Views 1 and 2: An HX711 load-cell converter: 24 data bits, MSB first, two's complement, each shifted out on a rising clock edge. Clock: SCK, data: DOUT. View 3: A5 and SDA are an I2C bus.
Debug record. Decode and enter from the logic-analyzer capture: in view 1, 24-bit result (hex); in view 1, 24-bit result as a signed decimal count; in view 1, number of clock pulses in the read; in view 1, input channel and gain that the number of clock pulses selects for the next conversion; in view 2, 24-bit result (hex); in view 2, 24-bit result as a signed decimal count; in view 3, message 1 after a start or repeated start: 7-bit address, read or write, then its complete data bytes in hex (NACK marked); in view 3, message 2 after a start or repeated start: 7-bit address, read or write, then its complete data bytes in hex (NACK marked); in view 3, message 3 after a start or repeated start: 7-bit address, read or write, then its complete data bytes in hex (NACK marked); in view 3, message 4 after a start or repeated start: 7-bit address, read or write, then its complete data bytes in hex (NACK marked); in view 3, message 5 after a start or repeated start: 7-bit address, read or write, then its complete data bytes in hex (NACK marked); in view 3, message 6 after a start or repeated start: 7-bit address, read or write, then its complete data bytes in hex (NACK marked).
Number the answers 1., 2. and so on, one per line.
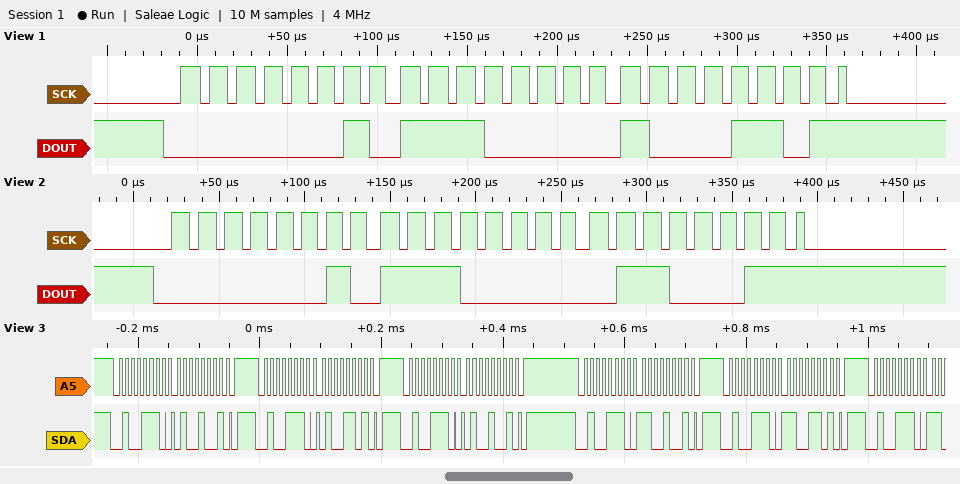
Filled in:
1. 0x02E08D
2. 188557
3. 25
4. channel A, gain 128
5. 0x02E063
6. 188515
7. 0x27 write: 49
8. 0x27 write: 4D
9. 0x27 write: 49
10. 0x27 write: C9
11. 0x27 write: CD
12. 0x27 write
